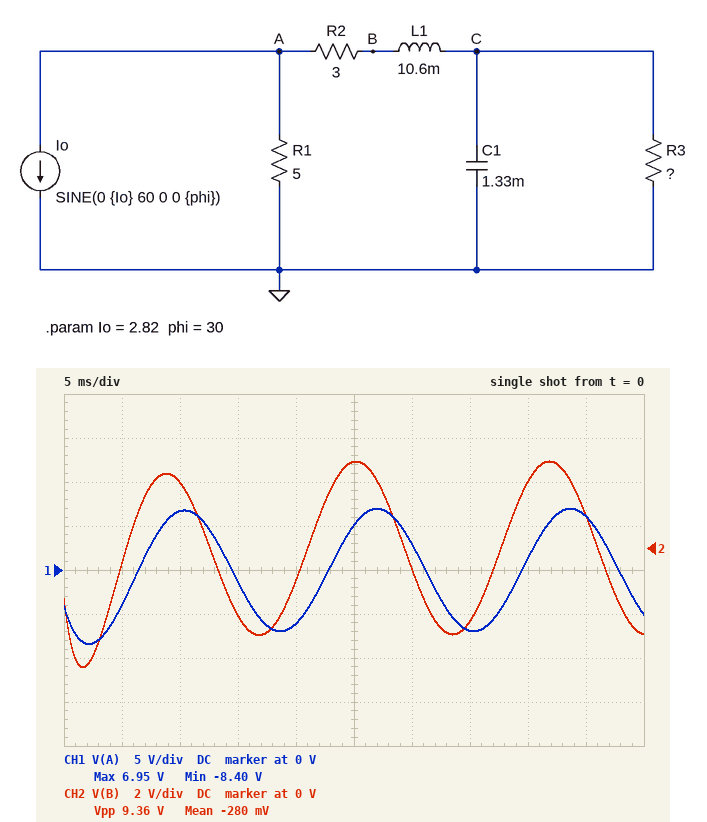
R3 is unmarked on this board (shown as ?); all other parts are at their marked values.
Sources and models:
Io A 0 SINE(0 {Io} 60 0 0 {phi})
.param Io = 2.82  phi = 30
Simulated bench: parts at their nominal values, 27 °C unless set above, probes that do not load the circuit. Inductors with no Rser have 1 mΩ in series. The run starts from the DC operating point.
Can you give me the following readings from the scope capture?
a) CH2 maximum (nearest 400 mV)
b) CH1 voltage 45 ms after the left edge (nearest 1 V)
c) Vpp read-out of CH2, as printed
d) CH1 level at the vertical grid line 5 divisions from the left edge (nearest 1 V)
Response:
4.0 V
6 V
9.36 V
5 V
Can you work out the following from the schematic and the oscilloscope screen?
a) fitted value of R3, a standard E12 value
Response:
3.9 Ω
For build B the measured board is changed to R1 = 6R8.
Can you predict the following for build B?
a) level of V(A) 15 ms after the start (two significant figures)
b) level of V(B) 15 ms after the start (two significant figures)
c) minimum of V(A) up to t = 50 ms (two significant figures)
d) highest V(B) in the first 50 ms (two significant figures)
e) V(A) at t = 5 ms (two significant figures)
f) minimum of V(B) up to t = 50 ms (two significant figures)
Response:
-1.9 V
-3.7 V
-10 V
4.5 V
-4.3 V
-6.5 V
